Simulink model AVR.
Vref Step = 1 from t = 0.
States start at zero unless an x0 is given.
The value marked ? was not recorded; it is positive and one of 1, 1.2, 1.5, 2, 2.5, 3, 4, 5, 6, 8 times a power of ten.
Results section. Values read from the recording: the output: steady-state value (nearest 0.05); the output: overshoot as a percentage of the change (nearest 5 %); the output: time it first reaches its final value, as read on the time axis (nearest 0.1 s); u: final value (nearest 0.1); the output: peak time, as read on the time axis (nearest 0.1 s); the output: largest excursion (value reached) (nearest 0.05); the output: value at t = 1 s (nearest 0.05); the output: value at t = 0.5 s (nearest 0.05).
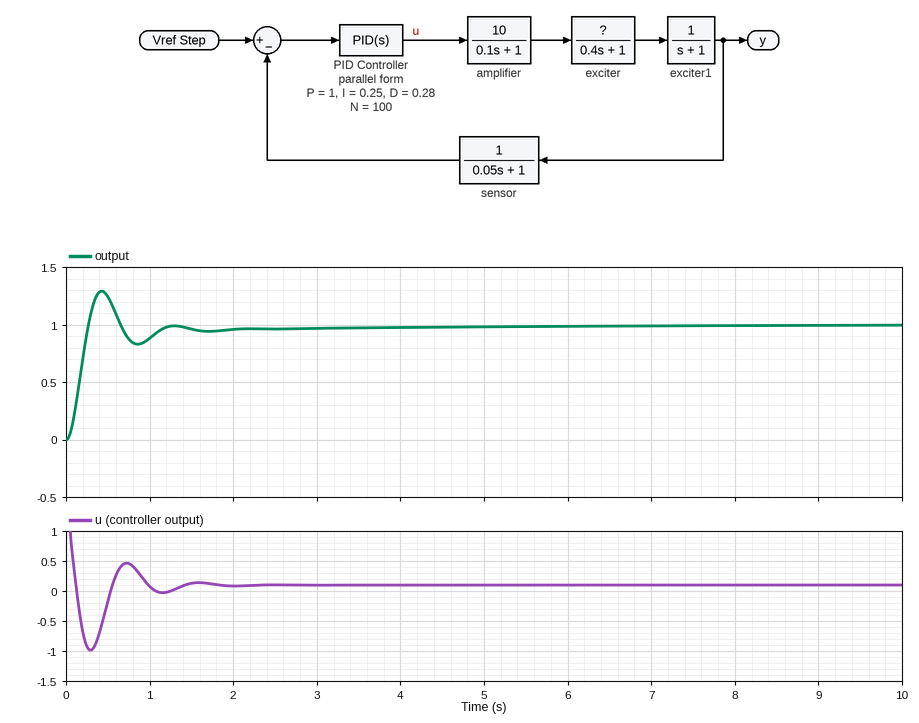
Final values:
1.00
30 %
0.3 s
0.1
0.4 s
1.30
0.90
1.25
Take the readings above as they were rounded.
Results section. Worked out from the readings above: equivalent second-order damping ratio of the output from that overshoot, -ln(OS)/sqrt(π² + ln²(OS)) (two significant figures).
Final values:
0.36
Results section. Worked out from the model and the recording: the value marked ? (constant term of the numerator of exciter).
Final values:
1
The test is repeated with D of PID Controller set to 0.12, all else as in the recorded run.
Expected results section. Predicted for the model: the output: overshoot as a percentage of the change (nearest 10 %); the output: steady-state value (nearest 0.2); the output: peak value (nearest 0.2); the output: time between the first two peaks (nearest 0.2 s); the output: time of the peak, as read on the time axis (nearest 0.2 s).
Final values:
40 %
1.0
1.4
1.2 s
0.6 s
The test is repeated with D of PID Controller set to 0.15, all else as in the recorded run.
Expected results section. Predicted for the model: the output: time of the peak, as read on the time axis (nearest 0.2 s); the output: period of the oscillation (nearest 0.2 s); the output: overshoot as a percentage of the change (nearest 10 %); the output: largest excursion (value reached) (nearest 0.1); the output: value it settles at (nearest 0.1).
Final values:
0.6 s
1.2 s
40 %
1.4
1.0
